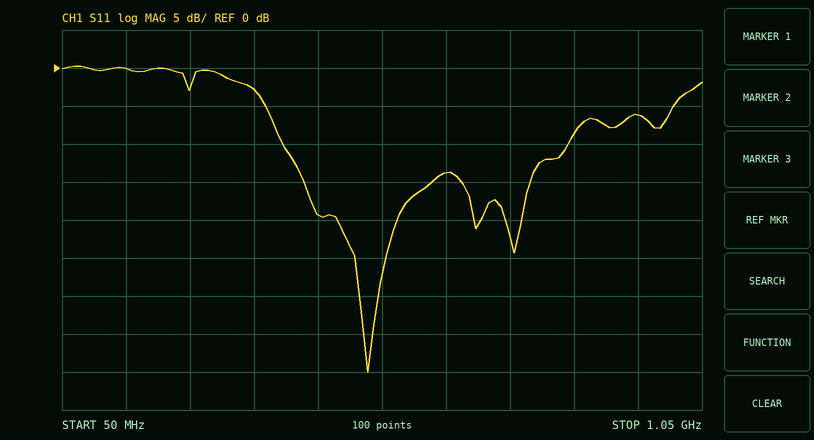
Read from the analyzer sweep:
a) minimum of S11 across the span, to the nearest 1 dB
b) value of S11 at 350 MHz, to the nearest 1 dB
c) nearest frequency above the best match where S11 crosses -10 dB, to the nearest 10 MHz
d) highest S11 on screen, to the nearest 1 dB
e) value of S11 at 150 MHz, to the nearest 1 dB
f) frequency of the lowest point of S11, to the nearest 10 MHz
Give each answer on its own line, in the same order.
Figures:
-40 dB
-3 dB
840 MHz
0 dB
0 dB
530 MHz
